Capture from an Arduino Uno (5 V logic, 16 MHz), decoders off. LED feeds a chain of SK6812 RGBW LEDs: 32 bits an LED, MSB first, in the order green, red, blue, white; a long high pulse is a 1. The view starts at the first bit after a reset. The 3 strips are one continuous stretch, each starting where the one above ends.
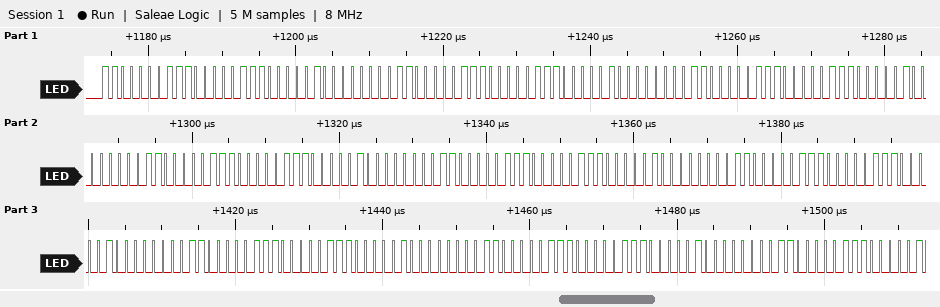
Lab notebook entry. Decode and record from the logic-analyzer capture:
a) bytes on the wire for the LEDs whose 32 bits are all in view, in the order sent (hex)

C1 C1 C1 00 C1 C1 C1 00 C1 C1 C1 00 C1 C1 C1 00 C1 C1 C1 00 C1 C1 C1 00 C1 C1 C1 00 C1 C1 C1 00
